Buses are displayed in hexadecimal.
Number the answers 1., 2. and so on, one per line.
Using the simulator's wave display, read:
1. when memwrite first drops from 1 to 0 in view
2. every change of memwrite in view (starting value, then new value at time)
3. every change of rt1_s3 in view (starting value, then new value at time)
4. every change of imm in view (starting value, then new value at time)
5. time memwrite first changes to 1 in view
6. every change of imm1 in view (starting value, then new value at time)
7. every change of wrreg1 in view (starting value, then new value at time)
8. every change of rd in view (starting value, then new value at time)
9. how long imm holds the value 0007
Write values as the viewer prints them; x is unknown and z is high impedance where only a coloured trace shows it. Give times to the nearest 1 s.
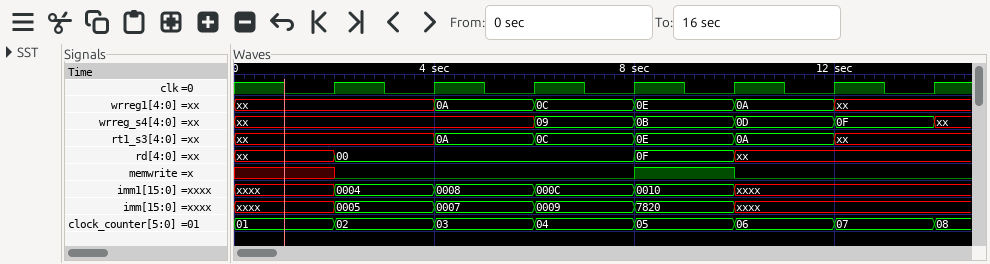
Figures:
1. 10 s
2. x, 0 at 2 s, 1 at 8 s, 0 at 10 s
3. xx, 0A at 4 s, 0C at 6 s, 0E at 8 s, 0A at 10 s, xx at 12 s
4. xxxx, 0005 at 2 s, 0007 at 4 s, 0009 at 6 s, 7820 at 8 s, xxxx at 10 s
5. 8 s
6. xxxx, 0004 at 2 s, 0008 at 4 s, 000C at 6 s, 0010 at 8 s, xxxx at 10 s
7. xx, 0A at 4 s, 0C at 6 s, 0E at 8 s, 0A at 10 s, xx at 12 s
8. xx, 00 at 2 s, 0F at 8 s, xx at 10 s
9. 2 s
